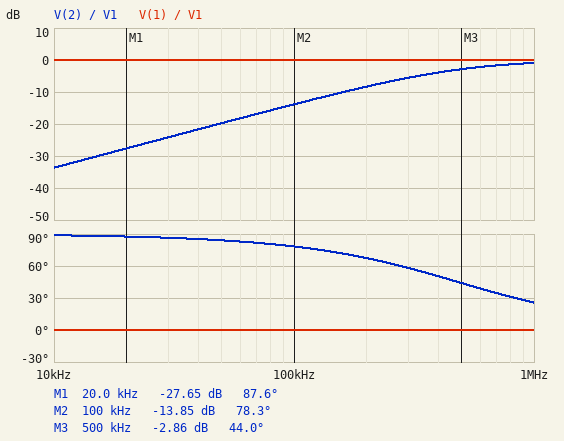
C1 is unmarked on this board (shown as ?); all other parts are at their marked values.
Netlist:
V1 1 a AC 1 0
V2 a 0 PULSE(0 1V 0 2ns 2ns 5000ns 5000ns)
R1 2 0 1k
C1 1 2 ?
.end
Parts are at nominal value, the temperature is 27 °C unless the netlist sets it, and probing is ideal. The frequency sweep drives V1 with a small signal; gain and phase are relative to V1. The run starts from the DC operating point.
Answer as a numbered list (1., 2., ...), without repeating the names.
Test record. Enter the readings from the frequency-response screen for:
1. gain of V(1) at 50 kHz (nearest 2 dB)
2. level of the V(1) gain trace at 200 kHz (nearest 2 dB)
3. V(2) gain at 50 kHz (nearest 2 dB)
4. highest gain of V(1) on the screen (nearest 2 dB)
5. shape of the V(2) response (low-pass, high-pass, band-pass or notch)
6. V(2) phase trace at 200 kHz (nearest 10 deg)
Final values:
1. 0 dB
2. 0 dB
3. -20 dB
4. 0 dB
5. high-pass
6. 70 deg
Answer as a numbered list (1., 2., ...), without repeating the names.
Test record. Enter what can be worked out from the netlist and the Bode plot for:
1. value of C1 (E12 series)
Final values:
1. 330 pF
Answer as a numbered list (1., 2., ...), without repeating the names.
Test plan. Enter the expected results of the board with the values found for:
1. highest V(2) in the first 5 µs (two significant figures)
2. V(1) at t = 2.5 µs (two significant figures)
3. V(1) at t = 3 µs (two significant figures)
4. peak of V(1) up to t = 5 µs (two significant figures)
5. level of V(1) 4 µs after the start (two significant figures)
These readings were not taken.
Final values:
1. 1.0 V
2. 1.0 V
3. 1.0 V
4. 1.0 V
5. 1.0 V
